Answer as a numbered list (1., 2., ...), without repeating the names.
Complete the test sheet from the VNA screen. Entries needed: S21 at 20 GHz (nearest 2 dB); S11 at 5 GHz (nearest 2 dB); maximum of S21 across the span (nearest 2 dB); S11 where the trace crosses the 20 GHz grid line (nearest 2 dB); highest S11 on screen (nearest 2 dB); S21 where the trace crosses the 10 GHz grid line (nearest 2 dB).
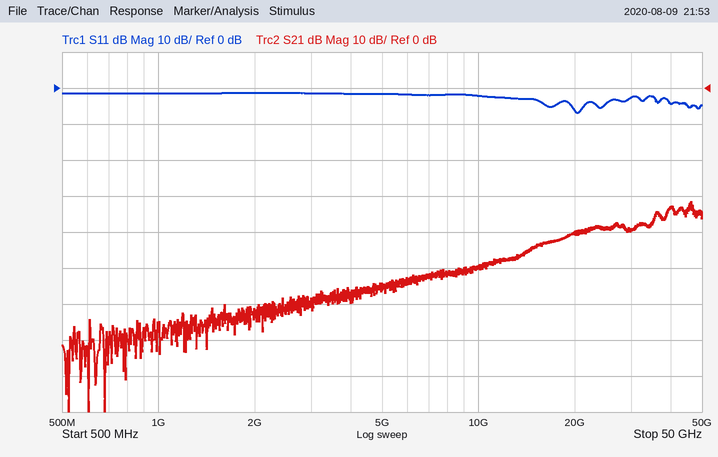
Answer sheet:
1. -40 dB
2. -2 dB
3. -32 dB
4. -6 dB
5. -2 dB
6. -50 dB
